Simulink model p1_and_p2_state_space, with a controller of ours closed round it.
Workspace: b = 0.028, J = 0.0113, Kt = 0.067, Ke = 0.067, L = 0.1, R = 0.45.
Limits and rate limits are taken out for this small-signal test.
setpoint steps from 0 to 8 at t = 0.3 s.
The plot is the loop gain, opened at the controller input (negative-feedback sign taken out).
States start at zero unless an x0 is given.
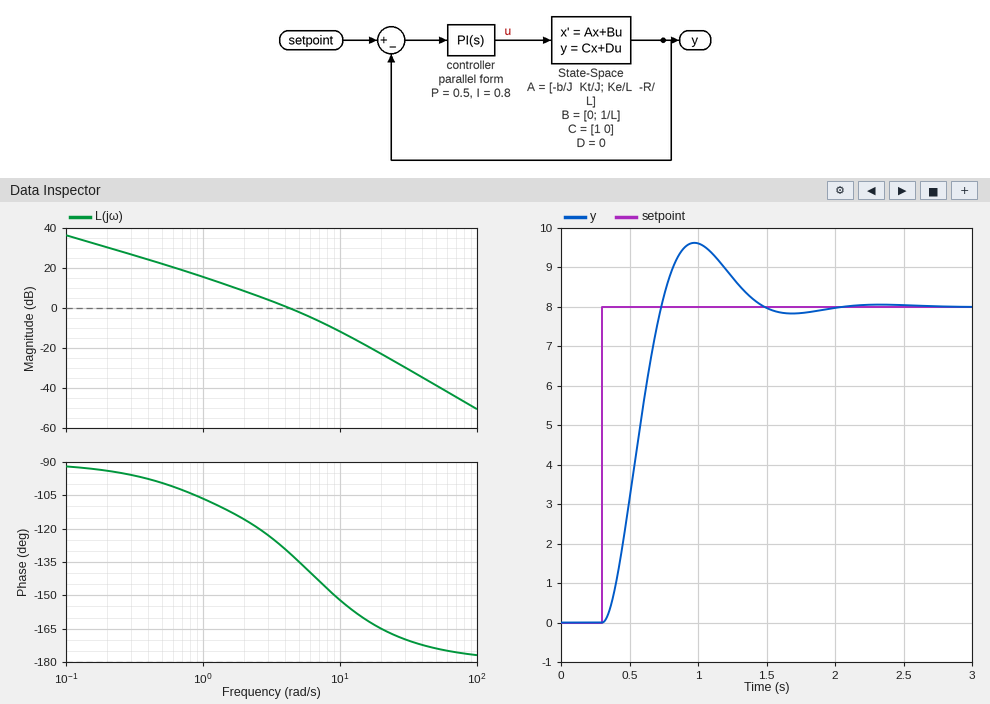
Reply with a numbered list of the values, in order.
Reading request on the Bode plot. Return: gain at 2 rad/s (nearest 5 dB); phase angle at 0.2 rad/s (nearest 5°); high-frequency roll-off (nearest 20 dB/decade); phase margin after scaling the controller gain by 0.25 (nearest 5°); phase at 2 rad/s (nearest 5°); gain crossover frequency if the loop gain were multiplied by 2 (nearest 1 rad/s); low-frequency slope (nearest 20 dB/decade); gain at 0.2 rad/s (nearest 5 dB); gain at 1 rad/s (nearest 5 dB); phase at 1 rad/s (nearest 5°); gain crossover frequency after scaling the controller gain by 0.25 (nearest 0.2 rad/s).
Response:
1. 10 dB
2. -95°
3. -40 dB/decade
4. 70°
5. -115°
6. 7 rad/s
7. -20 dB/decade
8. 30 dB
9. 15 dB
10. -105°
11. 1.4 rad/s
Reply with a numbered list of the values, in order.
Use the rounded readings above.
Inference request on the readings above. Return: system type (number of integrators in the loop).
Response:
1. 1
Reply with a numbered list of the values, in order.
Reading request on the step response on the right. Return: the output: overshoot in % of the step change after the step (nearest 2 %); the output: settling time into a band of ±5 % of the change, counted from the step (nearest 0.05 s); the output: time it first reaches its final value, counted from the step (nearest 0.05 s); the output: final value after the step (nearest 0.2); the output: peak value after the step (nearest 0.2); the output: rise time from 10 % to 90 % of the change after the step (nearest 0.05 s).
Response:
1. 20 %
2. 1.05 s
3. 0.45 s
4. 8.0
5. 9.6
6. 0.30 s
